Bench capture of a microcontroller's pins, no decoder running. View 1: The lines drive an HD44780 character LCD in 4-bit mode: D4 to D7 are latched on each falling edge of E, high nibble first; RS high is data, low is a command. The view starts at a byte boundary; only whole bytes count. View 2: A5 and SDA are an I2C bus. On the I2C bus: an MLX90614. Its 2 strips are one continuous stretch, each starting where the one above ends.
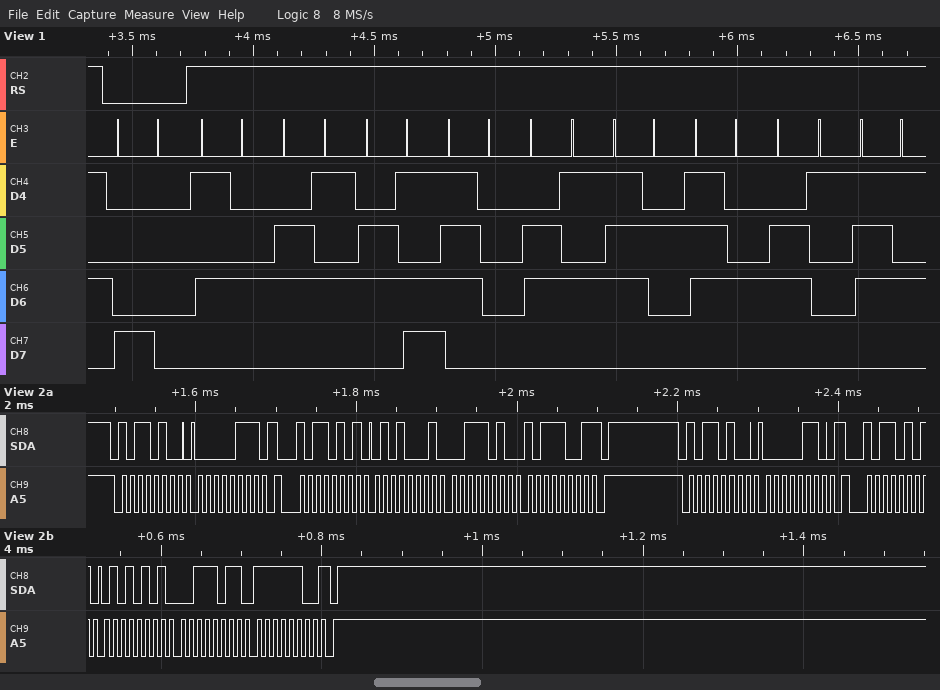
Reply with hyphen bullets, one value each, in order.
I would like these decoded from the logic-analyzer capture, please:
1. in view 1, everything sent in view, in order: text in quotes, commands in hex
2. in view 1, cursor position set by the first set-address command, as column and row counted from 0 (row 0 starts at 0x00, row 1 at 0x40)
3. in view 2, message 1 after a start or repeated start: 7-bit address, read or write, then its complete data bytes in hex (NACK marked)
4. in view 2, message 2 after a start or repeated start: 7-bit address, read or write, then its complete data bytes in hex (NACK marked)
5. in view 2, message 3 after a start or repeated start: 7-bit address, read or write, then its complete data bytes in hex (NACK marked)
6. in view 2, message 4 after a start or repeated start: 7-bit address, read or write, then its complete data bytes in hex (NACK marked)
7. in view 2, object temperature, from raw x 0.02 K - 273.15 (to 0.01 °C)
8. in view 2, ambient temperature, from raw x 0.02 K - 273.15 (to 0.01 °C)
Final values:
- 0x80 "Tempertau"
- column 0, row 0
- 0x5A write: 07
- 0x5A read: 51 3A B9 NACK
- 0x5A write: 06
- 0x5A read: 55 3B FC NACK
- 25.43 °C
- 30.63 °C
